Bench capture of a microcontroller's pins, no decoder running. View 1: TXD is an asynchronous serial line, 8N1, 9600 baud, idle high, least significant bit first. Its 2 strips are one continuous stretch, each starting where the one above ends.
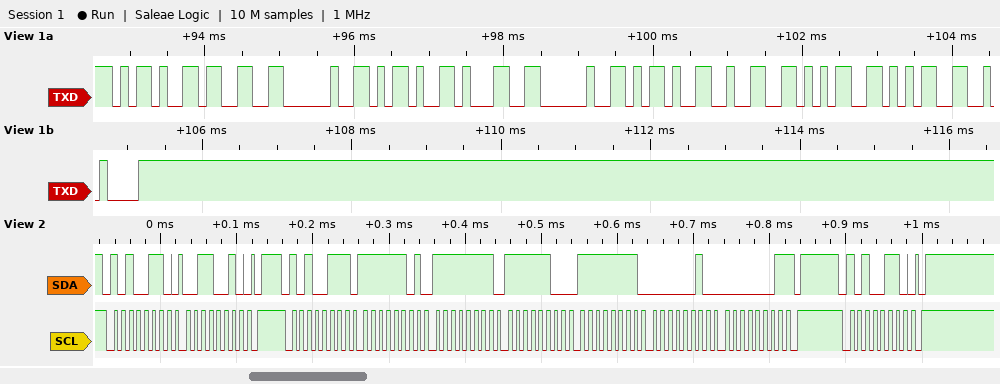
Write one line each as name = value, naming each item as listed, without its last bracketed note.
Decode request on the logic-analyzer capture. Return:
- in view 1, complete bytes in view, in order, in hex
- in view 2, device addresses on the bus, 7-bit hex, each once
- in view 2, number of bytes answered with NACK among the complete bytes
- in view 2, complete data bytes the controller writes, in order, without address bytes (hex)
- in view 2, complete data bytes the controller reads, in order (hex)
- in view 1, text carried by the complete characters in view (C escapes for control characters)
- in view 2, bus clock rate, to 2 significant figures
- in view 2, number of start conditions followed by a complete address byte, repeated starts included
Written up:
in view 1, complete bytes in view, in order, in hex = 0x2D 0x33 0x20 0x2D 0x31 0x20 0x2D 0x32 0x35 0x35 0x0A
in view 2, device addresses on the bus, 7-bit hex, each once = 0x53
in view 2, number of bytes answered with NACK among the complete bytes = 1
in view 2, complete data bytes the controller writes, in order, without address bytes = 32
in view 2, complete data bytes the controller reads, in order = FD FF FC FF 02 01
in view 1, text carried by the complete characters in view = "-3 -1 -255\n"
in view 2, bus clock rate, to 2 significant figures = 100 kHz
in view 2, number of start conditions followed by a complete address byte, repeated starts included = 3
